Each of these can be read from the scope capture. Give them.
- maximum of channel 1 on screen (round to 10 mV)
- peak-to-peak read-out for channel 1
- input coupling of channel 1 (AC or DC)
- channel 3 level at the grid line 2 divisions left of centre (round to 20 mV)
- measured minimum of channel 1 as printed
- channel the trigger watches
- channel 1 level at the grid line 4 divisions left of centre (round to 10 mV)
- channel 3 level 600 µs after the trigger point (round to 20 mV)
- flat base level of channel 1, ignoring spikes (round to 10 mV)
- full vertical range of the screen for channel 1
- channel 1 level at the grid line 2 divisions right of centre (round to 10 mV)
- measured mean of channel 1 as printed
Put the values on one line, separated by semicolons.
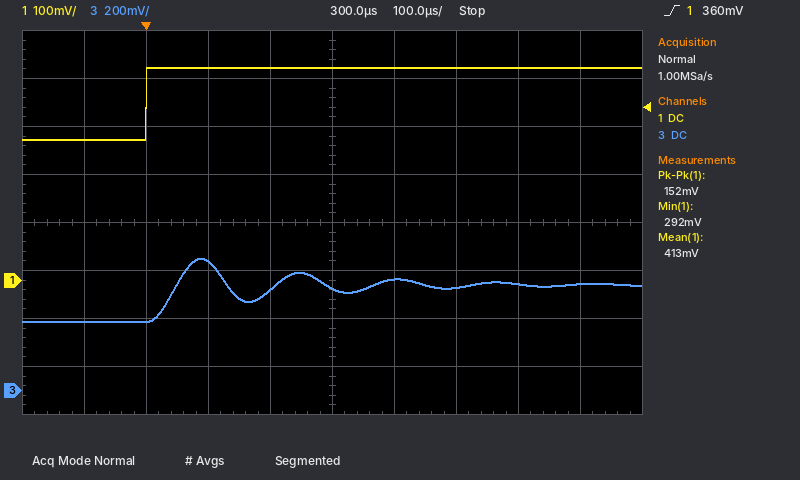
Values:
440 mV; 152 mV; DC; 540 mV; 292 mV; channel 1; 290 mV; 440 mV; 290 mV; 800 mV; 440 mV; 413 mV
